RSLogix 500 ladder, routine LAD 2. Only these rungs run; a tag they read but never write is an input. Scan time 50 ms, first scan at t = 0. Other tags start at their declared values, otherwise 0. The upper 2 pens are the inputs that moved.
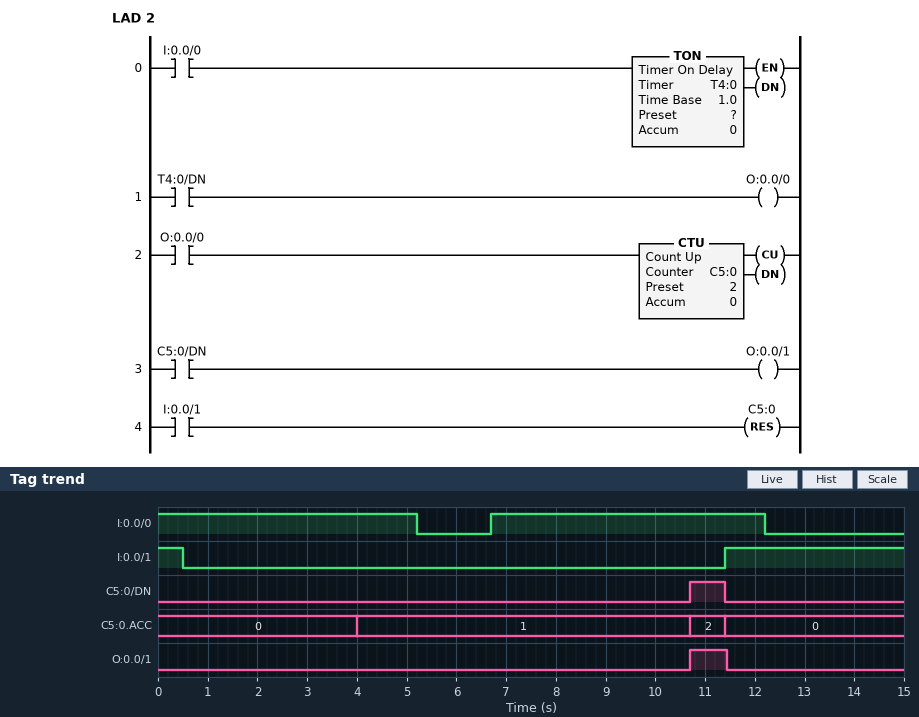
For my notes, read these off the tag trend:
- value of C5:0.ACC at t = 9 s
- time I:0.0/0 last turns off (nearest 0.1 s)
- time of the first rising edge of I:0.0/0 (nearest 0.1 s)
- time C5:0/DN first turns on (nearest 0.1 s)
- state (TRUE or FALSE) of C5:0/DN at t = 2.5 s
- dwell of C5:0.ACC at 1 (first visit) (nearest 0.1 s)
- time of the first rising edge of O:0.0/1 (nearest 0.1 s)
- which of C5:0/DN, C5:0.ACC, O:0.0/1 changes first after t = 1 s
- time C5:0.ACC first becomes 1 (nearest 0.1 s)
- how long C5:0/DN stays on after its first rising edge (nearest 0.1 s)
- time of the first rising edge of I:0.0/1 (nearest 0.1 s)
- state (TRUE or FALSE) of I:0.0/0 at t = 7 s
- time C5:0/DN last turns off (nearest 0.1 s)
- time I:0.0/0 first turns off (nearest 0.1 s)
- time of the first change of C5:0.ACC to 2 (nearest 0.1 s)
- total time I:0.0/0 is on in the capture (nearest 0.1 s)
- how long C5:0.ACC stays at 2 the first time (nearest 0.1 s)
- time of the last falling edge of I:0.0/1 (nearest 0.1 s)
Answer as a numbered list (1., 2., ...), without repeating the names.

1. 1
2. 12.2 s
3. 6.7 s
4. 10.7 s
5. FALSE
6. 6.7 s
7. 10.7 s
8. C5:0.ACC
9. 4.0 s
10. 0.7 s
11. 11.4 s
12. TRUE
13. 11.4 s
14. 5.2 s
15. 10.7 s
16. 10.7 s
17. 0.7 s
18. 0.5 s
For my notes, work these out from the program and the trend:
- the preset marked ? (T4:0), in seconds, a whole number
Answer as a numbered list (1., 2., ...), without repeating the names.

1. 4 s
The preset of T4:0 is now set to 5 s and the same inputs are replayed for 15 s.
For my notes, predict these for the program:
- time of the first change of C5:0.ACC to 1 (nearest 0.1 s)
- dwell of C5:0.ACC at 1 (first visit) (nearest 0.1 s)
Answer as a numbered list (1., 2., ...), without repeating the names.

1. 5.0 s
2. 6.4 s
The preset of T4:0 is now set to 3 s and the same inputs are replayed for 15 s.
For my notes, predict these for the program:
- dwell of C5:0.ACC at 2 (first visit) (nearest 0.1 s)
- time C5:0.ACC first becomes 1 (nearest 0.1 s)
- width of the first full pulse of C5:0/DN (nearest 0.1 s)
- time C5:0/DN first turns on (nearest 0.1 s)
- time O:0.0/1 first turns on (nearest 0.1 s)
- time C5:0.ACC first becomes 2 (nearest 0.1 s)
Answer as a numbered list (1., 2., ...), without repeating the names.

1. 1.7 s
2. 3.0 s
3. 1.7 s
4. 9.7 s
5. 9.7 s
6. 9.7 s
